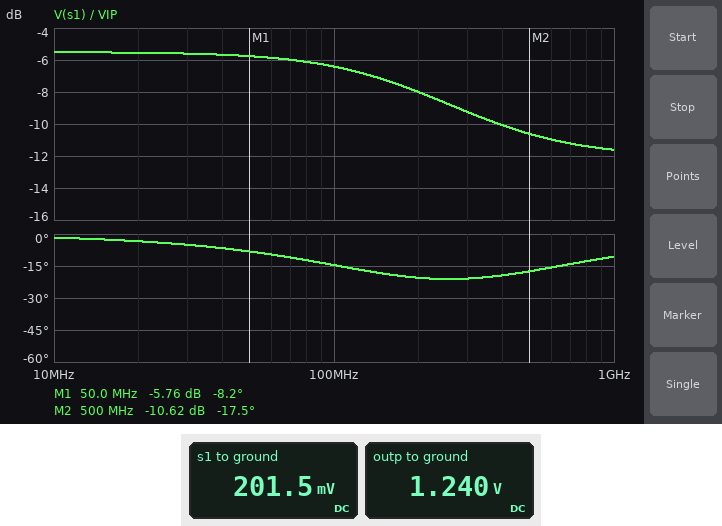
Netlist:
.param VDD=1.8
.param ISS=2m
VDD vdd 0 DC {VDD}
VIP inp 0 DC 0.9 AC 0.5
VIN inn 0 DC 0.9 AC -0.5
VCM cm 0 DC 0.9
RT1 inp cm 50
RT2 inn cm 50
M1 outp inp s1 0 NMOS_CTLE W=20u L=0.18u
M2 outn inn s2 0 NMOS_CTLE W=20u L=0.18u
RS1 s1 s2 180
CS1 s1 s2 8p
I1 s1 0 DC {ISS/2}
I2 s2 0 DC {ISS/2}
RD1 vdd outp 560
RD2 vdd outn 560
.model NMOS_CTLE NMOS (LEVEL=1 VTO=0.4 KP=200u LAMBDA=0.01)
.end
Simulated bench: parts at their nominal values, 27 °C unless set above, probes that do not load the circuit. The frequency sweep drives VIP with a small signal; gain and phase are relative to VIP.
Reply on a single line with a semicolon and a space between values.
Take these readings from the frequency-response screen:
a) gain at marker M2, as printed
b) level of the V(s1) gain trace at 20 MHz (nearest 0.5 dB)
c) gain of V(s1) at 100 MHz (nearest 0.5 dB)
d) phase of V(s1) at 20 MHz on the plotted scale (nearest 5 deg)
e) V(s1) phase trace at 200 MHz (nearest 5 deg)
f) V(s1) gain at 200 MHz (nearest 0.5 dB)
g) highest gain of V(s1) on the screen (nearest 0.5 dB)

-10.62 dB; -5.5 dB; -6.5 dB; -5 deg; -20 deg; -8.0 dB; -5.5 dB
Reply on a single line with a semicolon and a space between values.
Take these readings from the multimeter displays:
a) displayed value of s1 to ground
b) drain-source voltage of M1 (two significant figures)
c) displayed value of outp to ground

201.5 mV; 1.0 V; 1.240 V
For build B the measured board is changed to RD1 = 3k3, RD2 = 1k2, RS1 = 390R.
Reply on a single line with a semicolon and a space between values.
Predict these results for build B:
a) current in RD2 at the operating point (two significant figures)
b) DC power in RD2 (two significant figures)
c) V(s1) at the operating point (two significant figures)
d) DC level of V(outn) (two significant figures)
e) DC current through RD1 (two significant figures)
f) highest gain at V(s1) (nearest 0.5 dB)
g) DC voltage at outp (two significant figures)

1.4 mA; 2.4 mW; -190 mV; 110 mV; 590 µA; -21.5 dB; -150 mV
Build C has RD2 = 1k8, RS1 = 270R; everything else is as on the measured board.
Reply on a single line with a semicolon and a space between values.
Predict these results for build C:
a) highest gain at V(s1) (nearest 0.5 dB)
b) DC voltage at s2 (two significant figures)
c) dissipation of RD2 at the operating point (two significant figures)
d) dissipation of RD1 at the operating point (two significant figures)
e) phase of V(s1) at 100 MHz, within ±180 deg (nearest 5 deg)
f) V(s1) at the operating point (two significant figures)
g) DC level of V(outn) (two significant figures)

-1.0 dB; 140 mV; 1.3 mW; 740 µW; 0 deg; 180 mV; 270 mV
